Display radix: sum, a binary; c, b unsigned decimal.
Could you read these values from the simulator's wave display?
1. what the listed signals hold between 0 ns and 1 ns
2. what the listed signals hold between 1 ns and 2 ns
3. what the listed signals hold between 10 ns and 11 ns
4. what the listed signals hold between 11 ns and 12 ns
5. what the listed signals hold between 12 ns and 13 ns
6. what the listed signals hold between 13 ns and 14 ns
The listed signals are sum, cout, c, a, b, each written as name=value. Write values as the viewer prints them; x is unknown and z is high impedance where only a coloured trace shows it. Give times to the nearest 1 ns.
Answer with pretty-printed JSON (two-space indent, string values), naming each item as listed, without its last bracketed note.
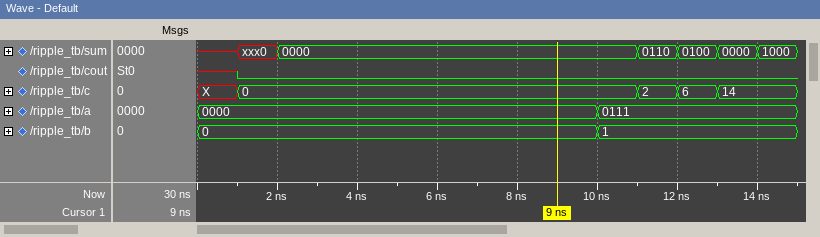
{
  "what the listed signals hold between 0 ns and 1 ns": "sum=x, cout=x, c=X, a=0000, b=0",
  "what the listed signals hold between 1 ns and 2 ns": "sum=xxx0, cout=0, c=0, a=0000, b=0",
  "what the listed signals hold between 10 ns and 11 ns": "sum=0000, cout=0, c=0, a=0111, b=1",
  "what the listed signals hold between 11 ns and 12 ns": "sum=0110, cout=0, c=2, a=0111, b=1",
  "what the listed signals hold between 12 ns and 13 ns": "sum=0100, cout=0, c=6, a=0111, b=1",
  "what the listed signals hold between 13 ns and 14 ns": "sum=0000, cout=0, c=14, a=0111, b=1"
}
